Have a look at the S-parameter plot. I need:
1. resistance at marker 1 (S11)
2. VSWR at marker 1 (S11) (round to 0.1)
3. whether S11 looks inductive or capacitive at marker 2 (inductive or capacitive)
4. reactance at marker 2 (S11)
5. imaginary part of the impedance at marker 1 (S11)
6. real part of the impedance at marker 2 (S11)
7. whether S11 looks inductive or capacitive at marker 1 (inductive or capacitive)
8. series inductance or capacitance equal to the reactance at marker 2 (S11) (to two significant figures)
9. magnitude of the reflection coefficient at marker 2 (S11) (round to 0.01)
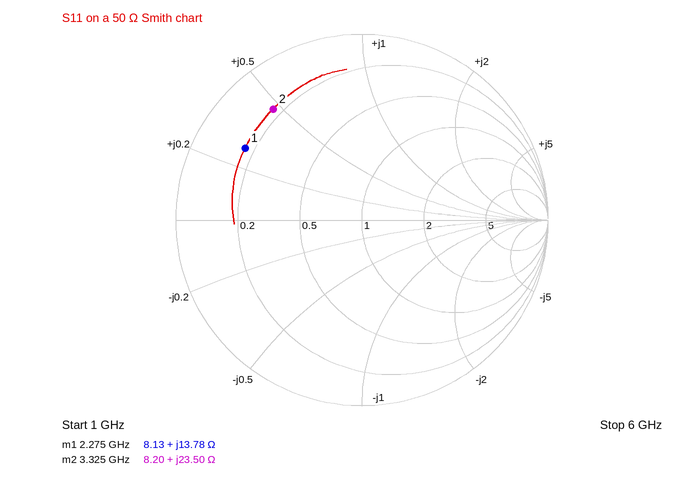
8.13 Ω
6.6
inductive
+23.50 Ω
+13.78 Ω
8.20 Ω
inductive
1.1 nH
0.76
